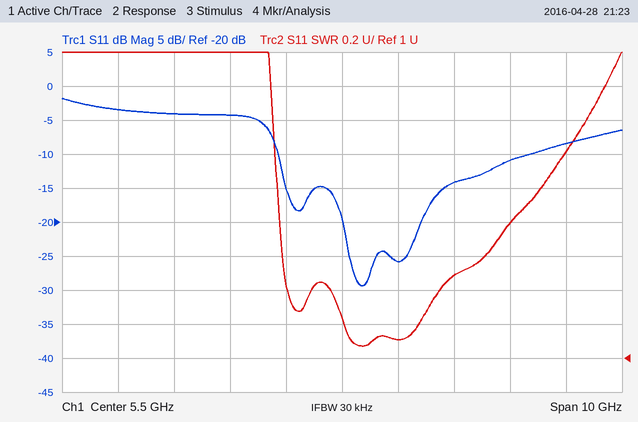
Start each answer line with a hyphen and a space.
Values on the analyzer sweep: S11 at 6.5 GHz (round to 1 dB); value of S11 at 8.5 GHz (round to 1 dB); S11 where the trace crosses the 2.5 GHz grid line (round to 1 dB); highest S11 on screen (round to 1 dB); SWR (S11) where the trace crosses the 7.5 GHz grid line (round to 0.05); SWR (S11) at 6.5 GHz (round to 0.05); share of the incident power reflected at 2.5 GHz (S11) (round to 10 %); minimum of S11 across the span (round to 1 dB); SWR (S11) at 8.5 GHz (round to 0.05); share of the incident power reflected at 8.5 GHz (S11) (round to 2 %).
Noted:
- -26 dB
- -11 dB
- -4 dB
- -2 dB
- 1.50
- 1.10
- 40 %
- -29 dB
- 1.80
- 8 %
